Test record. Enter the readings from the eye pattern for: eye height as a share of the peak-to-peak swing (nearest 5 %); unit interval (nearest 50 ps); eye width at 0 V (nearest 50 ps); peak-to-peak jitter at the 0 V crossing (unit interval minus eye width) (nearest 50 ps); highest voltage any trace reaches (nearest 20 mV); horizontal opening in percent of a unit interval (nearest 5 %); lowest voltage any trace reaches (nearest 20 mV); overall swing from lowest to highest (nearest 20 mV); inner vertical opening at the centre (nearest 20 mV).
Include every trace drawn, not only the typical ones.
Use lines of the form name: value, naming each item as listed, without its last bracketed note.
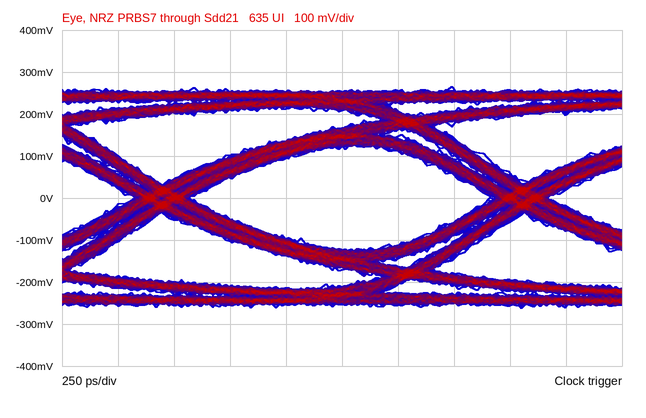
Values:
eye height as a share of the peak-to-peak swing: 45 %
unit interval: 1.60 ns
eye width at 0 V: 1.35 ns
peak-to-peak jitter at the 0 V crossing (unit interval minus eye width): 250 ps
highest voltage any trace reaches: 260 mV
horizontal opening in percent of a unit interval: 85 %
lowest voltage any trace reaches: -260 mV
overall swing from lowest to highest: 520 mV
inner vertical opening at the centre: 240 mV
